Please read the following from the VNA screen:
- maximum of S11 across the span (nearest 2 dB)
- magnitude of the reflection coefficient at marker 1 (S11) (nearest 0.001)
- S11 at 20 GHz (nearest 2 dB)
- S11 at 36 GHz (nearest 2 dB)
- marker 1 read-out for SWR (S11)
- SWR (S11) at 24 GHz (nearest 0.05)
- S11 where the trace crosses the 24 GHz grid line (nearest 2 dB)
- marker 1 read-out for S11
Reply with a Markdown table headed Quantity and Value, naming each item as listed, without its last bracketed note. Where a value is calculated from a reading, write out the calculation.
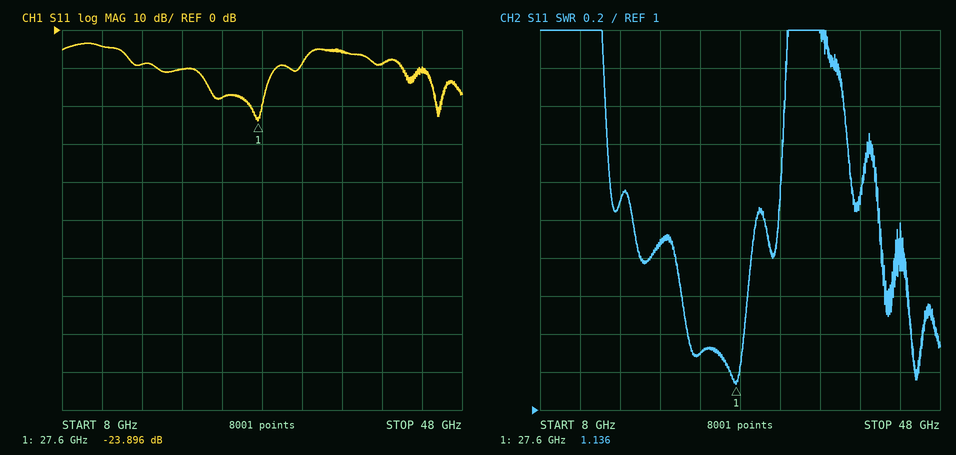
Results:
| Quantity | Value |
|---|---|
| maximum of S11 across the span | -4 dB |
| magnitude of the reflection coefficient at marker 1 (S11) | 10^(-23.896/20) ≈ 0.064 |
| S11 at 20 GHz | -10 dB |
| S11 at 36 GHz | -6 dB |
| marker 1 read-out for SWR | 1.136 |
| SWR (S11) at 24 GHz | 1.30 |
| S11 where the trace crosses the 24 GHz grid line | -18 dB |
| marker 1 read-out for S11 | -23.896 dB |
